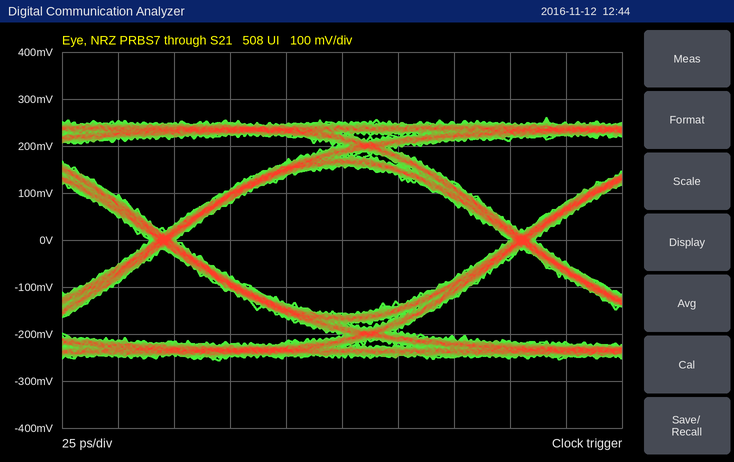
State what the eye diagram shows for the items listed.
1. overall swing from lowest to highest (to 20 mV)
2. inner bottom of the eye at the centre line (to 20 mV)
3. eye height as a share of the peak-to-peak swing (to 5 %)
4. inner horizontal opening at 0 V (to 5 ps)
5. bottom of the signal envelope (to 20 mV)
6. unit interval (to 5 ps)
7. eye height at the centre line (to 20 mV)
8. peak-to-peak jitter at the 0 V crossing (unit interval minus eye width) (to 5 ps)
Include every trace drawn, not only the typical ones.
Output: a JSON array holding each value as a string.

["520 mV", "-160 mV", "60 %", "150 ps", "-260 mV", "160 ps", "320 mV", "10 ps"]
